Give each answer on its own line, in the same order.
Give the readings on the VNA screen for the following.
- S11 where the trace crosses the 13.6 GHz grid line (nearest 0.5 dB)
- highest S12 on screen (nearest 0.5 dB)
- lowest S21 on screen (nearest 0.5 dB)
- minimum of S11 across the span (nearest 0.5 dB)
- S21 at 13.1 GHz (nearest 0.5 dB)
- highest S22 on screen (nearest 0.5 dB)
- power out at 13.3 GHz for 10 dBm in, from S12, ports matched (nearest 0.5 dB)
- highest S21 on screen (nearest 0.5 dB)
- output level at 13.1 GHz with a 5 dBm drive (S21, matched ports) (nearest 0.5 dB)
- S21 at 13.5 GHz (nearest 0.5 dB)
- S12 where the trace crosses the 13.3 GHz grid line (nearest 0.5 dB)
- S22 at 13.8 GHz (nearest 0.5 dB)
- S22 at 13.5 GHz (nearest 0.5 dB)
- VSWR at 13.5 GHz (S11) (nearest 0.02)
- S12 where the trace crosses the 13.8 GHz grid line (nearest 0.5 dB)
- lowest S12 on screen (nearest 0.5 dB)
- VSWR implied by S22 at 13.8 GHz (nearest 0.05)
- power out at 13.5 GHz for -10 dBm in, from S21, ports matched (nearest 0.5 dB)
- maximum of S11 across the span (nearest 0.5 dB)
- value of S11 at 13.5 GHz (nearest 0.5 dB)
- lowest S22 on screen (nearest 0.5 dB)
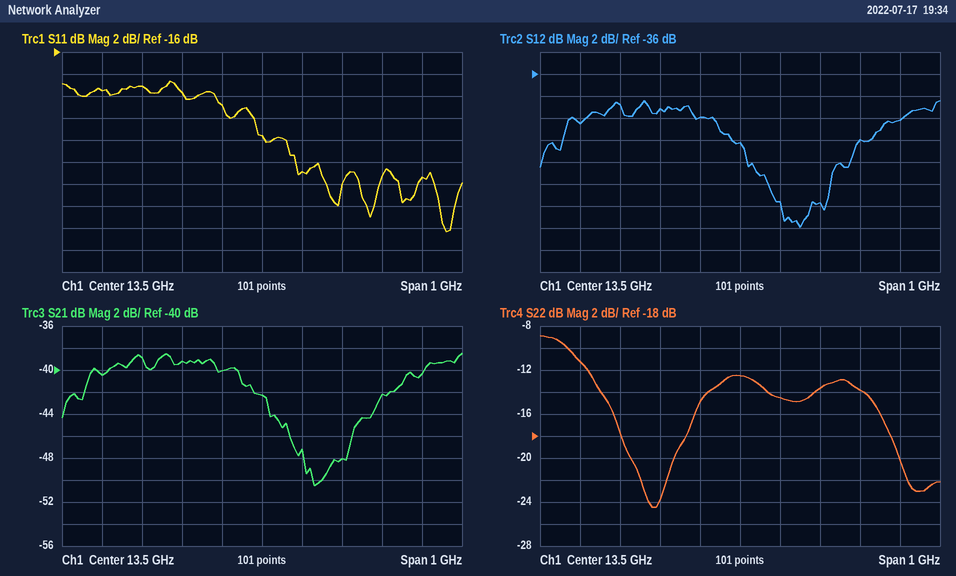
-27.0 dB
-38.5 dB
-50.5 dB
-32.5 dB
-40.5 dB
-9.0 dB
-29.0 dBm
-38.5 dB
-35.5 dBm
-42.5 dB
-39.0 dB
-14.0 dB
-12.5 dB
1.14
-42.0 dB
-50.0 dB
1.50
-52.5 dBm
-18.5 dB
-23.5 dB
-24.5 dB
